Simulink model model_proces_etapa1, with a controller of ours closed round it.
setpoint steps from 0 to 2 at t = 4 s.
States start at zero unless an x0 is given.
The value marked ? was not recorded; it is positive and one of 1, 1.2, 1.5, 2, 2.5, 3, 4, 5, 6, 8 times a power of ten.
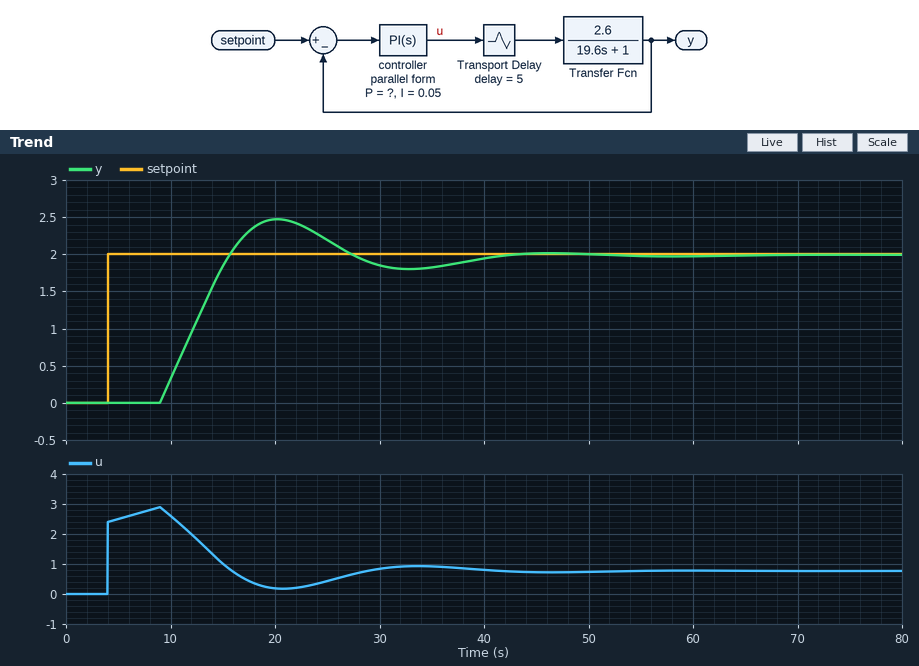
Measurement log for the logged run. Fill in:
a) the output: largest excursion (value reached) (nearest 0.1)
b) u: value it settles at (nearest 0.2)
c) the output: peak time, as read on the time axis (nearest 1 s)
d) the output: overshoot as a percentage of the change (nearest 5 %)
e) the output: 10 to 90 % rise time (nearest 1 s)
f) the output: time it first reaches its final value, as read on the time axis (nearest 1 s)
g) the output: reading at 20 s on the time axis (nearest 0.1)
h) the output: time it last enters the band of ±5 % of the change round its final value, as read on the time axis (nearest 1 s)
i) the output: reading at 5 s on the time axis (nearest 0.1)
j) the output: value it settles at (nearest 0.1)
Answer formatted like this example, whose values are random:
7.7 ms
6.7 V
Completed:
2.5
0.8
20 s
25 %
5 s
16 s
2.5
38 s
0.0
2.0
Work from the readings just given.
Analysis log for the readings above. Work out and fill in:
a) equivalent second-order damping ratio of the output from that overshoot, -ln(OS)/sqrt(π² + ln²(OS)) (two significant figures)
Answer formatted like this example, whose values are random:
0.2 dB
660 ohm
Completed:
0.40
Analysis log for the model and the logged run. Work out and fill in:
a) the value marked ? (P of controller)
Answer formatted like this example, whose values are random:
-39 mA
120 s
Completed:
1.2
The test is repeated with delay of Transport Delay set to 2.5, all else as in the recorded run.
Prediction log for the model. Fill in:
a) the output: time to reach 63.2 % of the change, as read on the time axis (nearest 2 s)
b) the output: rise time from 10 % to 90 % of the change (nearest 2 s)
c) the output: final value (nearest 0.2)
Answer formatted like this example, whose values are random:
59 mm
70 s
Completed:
10 s
8 s
2.0
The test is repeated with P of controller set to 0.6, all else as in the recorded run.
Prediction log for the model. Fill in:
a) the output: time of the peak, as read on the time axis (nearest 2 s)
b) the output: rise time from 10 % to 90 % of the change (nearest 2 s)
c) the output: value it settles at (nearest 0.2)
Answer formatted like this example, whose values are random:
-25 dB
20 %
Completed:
32 s
10 s
2.0
